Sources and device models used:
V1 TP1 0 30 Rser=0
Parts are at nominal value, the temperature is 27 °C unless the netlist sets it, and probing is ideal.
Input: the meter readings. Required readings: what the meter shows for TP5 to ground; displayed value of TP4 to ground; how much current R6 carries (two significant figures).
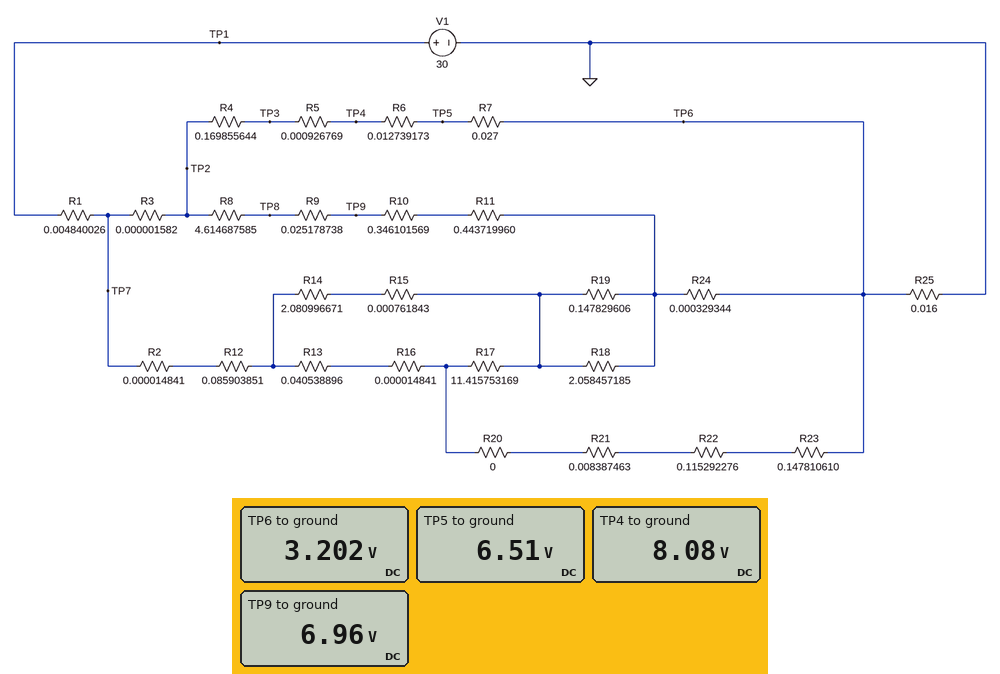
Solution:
6.51 V
8.08 V
120 A
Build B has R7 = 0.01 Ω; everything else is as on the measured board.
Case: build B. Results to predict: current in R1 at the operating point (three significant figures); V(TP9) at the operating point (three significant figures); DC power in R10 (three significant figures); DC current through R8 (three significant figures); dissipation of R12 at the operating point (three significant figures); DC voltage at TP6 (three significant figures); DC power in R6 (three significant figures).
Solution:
209 A
7.08 V
7.71 W
4.72 A
447 W
3.35 V
224 W
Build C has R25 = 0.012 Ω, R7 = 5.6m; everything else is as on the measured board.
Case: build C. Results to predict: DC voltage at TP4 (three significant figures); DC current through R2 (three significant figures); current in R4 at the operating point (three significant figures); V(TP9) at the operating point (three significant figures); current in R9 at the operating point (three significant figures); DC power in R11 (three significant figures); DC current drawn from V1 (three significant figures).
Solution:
5.17 V
74.1 A
139 A
6.45 V
4.85 A
10.4 W
218 A
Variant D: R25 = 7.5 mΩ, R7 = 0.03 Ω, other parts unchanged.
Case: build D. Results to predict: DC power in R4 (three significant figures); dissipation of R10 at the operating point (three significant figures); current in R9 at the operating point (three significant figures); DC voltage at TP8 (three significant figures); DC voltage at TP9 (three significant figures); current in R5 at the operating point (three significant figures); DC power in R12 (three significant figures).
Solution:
2.80 kW
8.81 W
5.05 A
5.70 V
5.57 V
128 A
511 W
